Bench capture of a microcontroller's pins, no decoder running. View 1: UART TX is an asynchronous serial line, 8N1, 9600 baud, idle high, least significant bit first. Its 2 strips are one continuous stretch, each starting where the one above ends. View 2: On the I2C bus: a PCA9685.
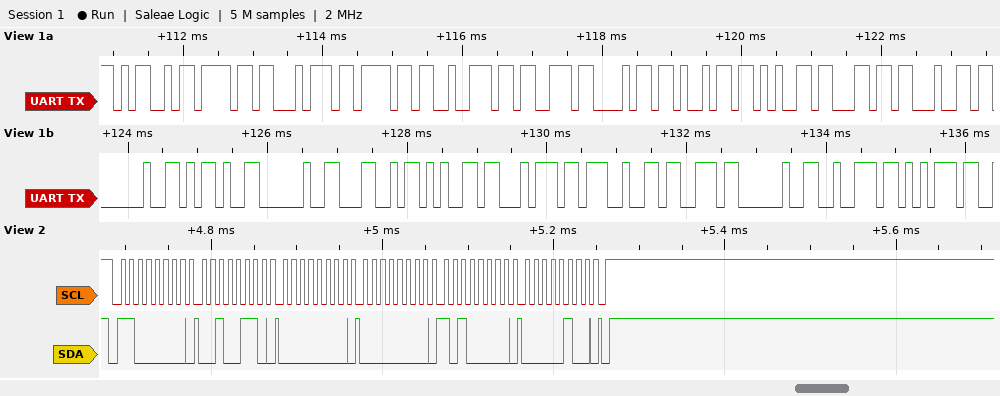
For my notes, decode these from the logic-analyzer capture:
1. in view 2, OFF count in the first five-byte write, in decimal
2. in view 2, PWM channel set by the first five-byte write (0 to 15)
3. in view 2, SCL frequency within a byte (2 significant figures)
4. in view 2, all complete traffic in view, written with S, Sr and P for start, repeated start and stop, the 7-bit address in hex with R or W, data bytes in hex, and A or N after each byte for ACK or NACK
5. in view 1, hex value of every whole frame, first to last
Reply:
1184
8
100 kHz
S 60W A 26 A 00 A 00 A A0 A 04 A P
0x4D 0x6F 0x74 0x6F 0x72 0x73 0x68 0x69 0x65 0x6C 0x64 0x20 0x2D 0x20 0x4C 0x65 0x74 0x27 0x73 0x20 0x72 0x75
